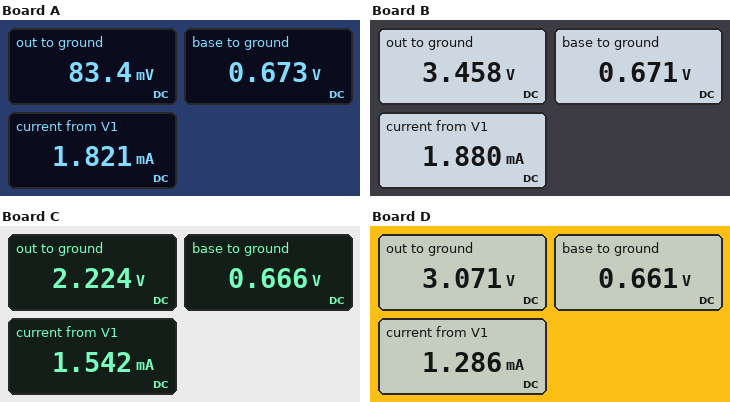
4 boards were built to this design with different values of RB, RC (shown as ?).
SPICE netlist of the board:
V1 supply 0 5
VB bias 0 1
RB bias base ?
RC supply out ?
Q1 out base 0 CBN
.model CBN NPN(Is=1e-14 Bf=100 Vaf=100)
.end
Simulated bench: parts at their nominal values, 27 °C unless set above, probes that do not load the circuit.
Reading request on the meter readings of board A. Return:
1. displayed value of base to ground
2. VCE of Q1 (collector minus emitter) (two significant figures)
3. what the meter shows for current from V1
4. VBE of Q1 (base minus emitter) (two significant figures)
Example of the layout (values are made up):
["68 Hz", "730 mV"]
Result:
["0.673 V", "83 mV", "1.821 mA", "670 mV"]
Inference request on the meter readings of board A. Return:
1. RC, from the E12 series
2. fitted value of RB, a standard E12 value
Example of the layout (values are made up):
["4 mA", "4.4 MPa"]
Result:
["2.7 kΩ", "3.3 kΩ"]
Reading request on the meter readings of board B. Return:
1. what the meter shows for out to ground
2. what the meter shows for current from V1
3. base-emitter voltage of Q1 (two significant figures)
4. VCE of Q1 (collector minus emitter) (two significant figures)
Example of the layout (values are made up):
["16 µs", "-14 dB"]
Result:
["3.458 V", "1.880 mA", "670 mV", "3.5 V"]
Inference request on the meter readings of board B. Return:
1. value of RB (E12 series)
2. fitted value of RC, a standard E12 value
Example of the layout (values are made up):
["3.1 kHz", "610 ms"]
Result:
["18 kΩ", "820 Ω"]
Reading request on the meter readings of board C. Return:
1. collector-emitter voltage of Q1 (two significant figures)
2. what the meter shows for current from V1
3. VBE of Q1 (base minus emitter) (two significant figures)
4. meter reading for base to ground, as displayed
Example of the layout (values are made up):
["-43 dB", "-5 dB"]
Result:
["2.2 V", "1.542 mA", "670 mV", "0.666 V"]
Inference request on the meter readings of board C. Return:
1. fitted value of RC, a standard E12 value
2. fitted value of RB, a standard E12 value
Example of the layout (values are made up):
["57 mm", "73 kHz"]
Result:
["1.8 kΩ", "22 kΩ"]
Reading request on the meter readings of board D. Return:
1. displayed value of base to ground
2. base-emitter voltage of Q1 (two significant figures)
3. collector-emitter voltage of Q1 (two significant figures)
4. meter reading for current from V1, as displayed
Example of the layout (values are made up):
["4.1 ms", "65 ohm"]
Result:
["0.661 V", "660 mV", "3.1 V", "1.286 mA"]
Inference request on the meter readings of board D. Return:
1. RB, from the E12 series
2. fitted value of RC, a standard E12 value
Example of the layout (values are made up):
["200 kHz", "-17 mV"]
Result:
["27 kΩ", "1.5 kΩ"]
